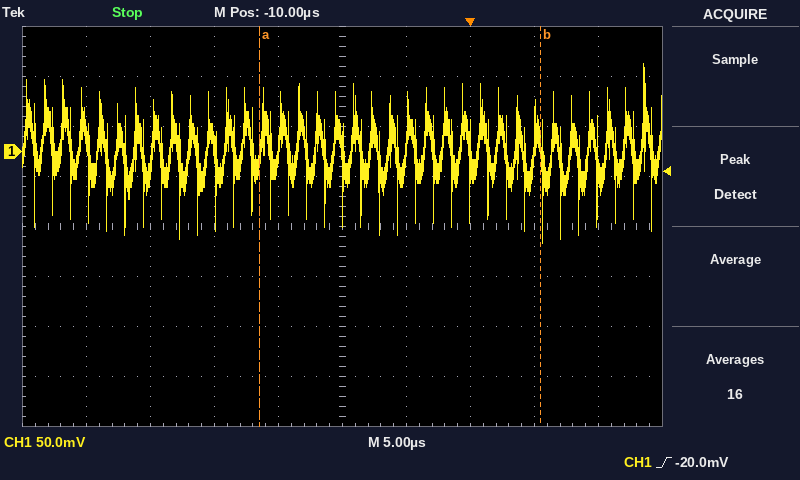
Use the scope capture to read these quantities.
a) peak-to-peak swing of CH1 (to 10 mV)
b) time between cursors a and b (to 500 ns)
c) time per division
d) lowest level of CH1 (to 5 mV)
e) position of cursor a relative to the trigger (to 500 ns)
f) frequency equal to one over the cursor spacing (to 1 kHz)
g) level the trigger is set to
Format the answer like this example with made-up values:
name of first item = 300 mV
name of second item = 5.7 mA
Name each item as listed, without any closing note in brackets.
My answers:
peak-to-peak swing of CH1 = 180 mV
time between cursors a and b = 22.0 µs
time per division = 5 µs
lowest level of CH1 = -90 mV
position of cursor a relative to the trigger = -16.5 µs
frequency equal to one over the cursor spacing = 45 kHz
level the trigger is set to = -20.0 mV
